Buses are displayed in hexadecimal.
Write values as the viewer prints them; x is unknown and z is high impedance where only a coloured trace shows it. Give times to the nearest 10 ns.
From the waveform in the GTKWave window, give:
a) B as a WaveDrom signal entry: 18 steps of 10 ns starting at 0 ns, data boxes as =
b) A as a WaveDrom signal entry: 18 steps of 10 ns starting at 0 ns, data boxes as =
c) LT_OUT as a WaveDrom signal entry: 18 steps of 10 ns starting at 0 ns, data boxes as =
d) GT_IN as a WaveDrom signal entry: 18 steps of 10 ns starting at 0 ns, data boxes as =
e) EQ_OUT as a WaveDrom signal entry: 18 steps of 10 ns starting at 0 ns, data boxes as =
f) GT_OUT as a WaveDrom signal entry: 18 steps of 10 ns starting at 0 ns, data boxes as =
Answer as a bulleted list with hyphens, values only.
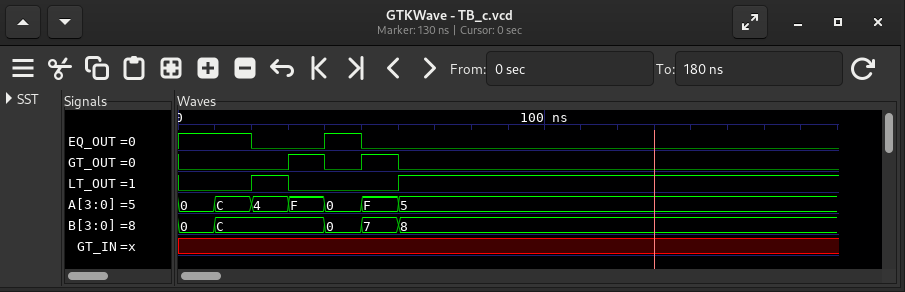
- {name: 'B', wave: '==..===...........', data: '0 C 0 7 8'}
- {name: 'A', wave: '=======...........', data: '0 C 4 F 0 F 5'}
- {name: 'LT_OUT', wave: '0.10..1...........'}
- {name: 'GT_IN', wave: 'x.................'}
- {name: 'EQ_OUT', wave: '1.0.10............'}
- {name: 'GT_OUT', wave: '0..1010...........'}
